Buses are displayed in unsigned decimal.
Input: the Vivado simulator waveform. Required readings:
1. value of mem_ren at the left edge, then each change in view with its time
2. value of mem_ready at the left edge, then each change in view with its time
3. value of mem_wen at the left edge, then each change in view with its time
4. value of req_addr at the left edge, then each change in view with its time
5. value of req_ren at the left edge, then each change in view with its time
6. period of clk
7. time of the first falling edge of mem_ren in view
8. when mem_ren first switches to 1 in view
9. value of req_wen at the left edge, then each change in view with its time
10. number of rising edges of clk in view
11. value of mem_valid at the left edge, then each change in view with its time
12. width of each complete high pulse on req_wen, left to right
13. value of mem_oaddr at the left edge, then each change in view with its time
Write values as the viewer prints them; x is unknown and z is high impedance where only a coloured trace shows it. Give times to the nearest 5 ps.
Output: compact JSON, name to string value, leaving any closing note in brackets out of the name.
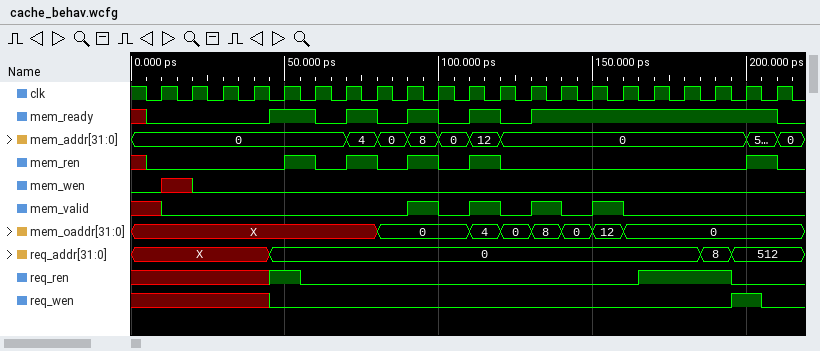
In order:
{"value of mem_ren at the left edge, then each change in view with its time": "x, 0 at 5 ps, 1 at 50 ps, 0 at 60 ps, 1 at 70 ps, 0 at 80 ps, 1 at 90 ps, 0 at 100 ps, 1 at 110 ps, 0 at 120 ps, 1 at 200 ps, 0 at 210 ps", "value of mem_ready at the left edge, then each change in view with its time": "x, 0 at 5 ps, 1 at 45 ps, 0 at 60 ps, 1 at 70 ps, 0 at 80 ps, 1 at 90 ps, 0 at 100 ps, 1 at 110 ps, 0 at 120 ps, 1 at 130 ps, 0 at 210 ps", "value of mem_wen at the left edge, then each change in view with its time": "0, x at 10 ps, 0 at 20 ps", "value of req_addr at the left edge, then each change in view with its time": "X, 0 at 45 ps, 8 at 185 ps, 512 at 195 ps", "value of req_ren at the left edge, then each change in view with its time": "x, 1 at 45 ps, 0 at 55 ps, 1 at 165 ps, 0 at 195 ps", "period of clk": "10 ps", "time of the first falling edge of mem_ren in view": "60 ps", "when mem_ren first switches to 1 in view": "50 ps", "value of req_wen at the left edge, then each change in view with its time": "x, 0 at 45 ps, 1 at 195 ps, 0 at 205 ps", "number of rising edges of clk in view": "21", "value of mem_valid at the left edge, then each change in view with its time": "x, 0 at 10 ps, 1 at 90 ps, 0 at 100 ps, 1 at 110 ps, 0 at 120 ps, 1 at 130 ps, 0 at 140 ps, 1 at 150 ps, 0 at 160 ps", "width of each complete high pulse on req_wen, left to right": "10 ps", "value of mem_oaddr at the left edge, then each change in view with its time": "X, 0 at 80 ps, 4 at 110 ps, 0 at 120 ps, 8 at 130 ps, 0 at 140 ps, 12 at 150 ps, 0 at 160 ps"}
